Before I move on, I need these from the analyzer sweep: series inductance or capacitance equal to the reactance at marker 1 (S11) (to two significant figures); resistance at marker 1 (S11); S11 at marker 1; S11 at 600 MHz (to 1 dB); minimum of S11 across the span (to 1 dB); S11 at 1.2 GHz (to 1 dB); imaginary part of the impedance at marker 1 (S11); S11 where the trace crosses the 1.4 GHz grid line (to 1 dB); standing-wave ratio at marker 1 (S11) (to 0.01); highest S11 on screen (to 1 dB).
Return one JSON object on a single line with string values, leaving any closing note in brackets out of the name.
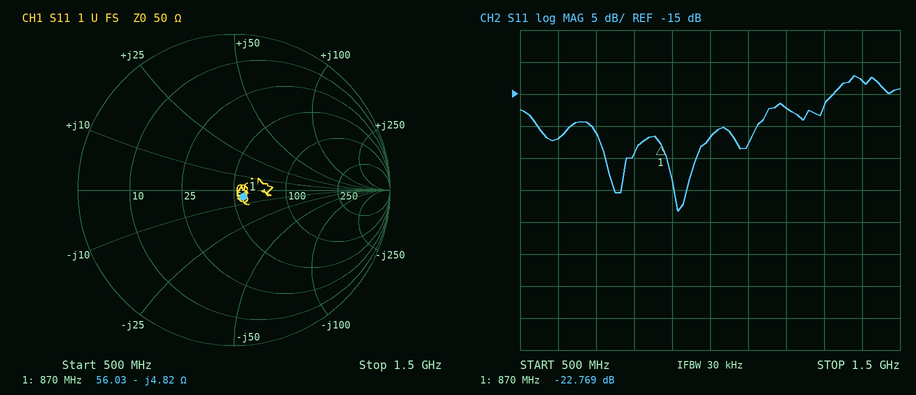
{"series inductance or capacitance equal to the reactance at marker 1 (S11)": "38 pF", "resistance at marker 1": "56.03 Ω", "S11 at marker 1": "-22.769 dB", "S11 at 600 MHz": "-22 dB", "minimum of S11 across the span": "-33 dB", "S11 at 1.2 GHz": "-17 dB", "imaginary part of the impedance at marker 1": "-4.82 Ω", "S11 where the trace crosses the 1.4 GHz grid line": "-13 dB", "standing-wave ratio at marker 1 (S11)": "1.16", "highest S11 on screen": "-12 dB"}
